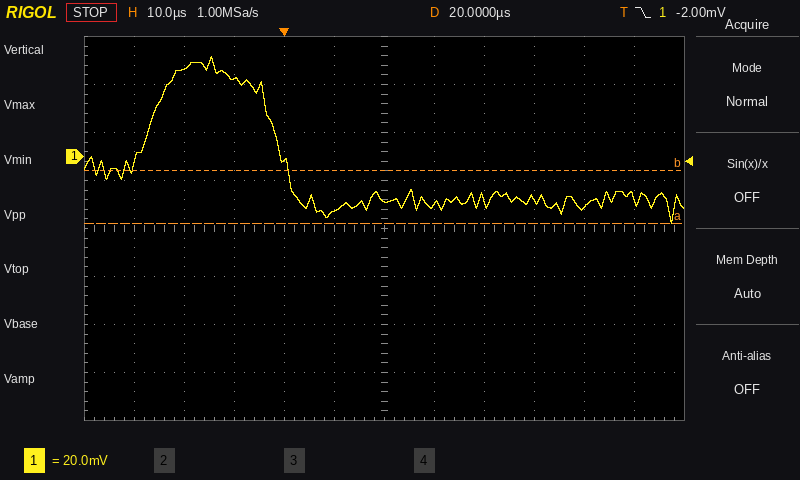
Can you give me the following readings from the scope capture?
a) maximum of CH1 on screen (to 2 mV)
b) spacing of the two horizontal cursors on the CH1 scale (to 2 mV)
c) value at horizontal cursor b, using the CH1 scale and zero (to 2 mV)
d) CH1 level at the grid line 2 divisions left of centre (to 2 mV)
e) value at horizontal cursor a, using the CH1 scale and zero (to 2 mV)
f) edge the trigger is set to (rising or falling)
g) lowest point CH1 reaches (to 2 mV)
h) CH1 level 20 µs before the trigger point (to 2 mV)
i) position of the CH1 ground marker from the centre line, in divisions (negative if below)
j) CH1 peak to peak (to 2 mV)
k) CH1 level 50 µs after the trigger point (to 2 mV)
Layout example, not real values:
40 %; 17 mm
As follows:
42 mV; 22 mV; -6 mV; -2 mV; -28 mV; falling; -28 mV; 36 mV; +1.5 div; 70 mV; -18 mV
